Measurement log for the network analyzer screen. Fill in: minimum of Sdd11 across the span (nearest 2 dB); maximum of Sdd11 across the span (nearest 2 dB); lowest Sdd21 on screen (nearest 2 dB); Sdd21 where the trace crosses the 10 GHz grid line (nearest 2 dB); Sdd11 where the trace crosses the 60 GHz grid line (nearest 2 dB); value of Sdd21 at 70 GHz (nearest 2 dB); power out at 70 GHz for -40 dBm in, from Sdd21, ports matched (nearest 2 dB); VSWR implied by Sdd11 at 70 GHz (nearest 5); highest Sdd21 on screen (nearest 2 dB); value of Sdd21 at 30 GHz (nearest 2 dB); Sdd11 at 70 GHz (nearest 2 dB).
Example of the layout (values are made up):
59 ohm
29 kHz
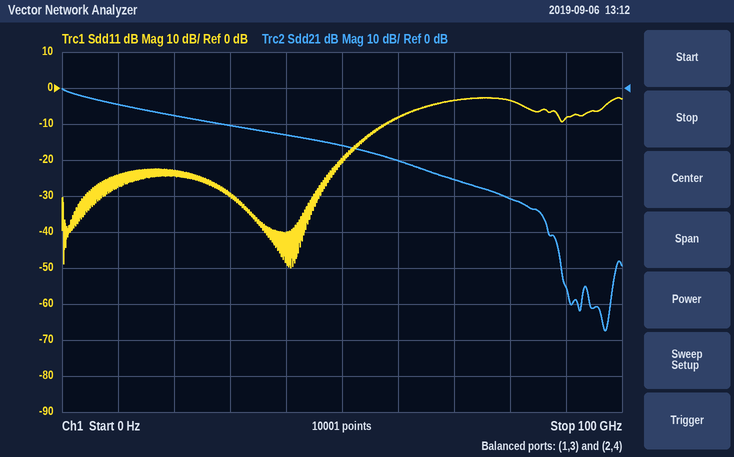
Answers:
-50 dB
-2 dB
-68 dB
-4 dB
-8 dB
-26 dB
-66 dBm
5
0 dB
-10 dB
-4 dB
